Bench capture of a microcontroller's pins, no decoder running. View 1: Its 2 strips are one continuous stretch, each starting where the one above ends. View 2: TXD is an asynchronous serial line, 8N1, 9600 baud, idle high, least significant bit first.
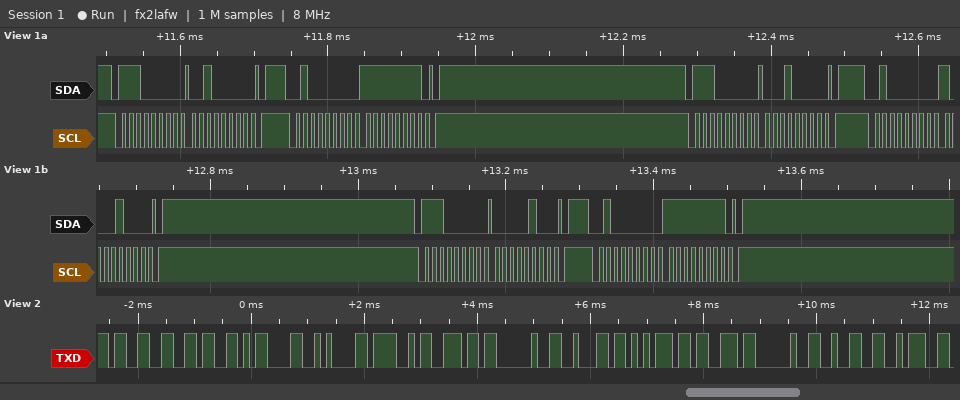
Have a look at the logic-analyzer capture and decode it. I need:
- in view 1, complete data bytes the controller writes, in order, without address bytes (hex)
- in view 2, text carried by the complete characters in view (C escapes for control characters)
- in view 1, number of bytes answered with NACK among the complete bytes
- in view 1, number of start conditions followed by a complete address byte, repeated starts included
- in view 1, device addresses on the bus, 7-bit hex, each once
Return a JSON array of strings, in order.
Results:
["20 FF 10 88 04 FF", "\"36\\r\\nOn bus 2:\"", "0", "6", "0x70 0x20"]
